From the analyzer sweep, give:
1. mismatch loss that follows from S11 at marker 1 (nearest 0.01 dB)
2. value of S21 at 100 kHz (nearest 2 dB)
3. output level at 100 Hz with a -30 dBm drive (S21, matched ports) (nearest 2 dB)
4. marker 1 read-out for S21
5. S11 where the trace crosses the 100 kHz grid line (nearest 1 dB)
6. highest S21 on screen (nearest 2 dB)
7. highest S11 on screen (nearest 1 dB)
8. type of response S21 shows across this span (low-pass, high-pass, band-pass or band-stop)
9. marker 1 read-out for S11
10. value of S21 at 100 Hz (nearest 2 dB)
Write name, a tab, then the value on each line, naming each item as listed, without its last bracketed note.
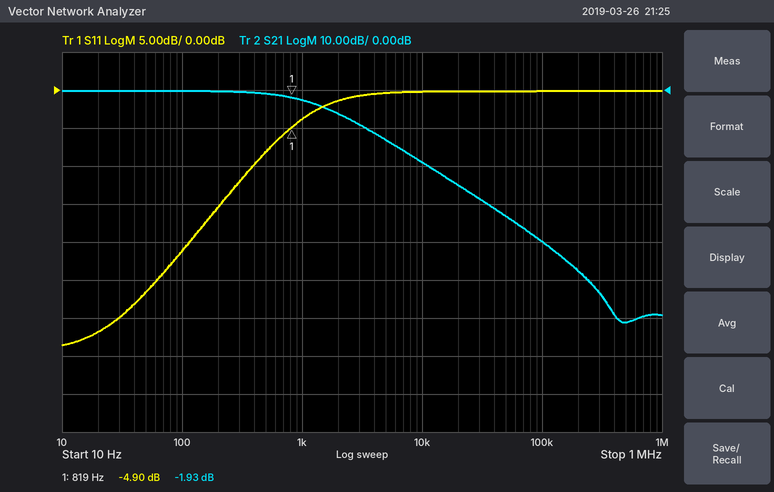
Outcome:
mismatch loss that follows from S11 at marker 1	1.70 dB
value of S21 at 100 kHz	-40 dB
output level at 100 Hz with a -30 dBm drive (S21, matched ports)	-30 dBm
marker 1 read-out for S21	-1.93 dB
S11 where the trace crosses the 100 kHz grid line	0 dB
highest S21 on screen	0 dB
highest S11 on screen	0 dB
type of response S21 shows across this span	low-pass
marker 1 read-out for S11	-4.90 dB
value of S21 at 100 Hz	0 dB
